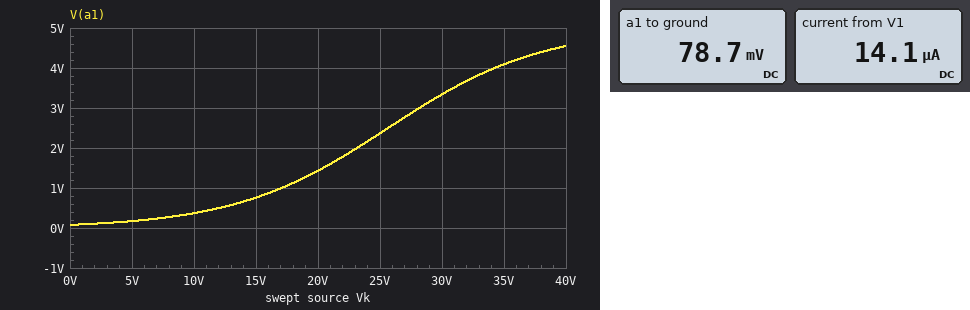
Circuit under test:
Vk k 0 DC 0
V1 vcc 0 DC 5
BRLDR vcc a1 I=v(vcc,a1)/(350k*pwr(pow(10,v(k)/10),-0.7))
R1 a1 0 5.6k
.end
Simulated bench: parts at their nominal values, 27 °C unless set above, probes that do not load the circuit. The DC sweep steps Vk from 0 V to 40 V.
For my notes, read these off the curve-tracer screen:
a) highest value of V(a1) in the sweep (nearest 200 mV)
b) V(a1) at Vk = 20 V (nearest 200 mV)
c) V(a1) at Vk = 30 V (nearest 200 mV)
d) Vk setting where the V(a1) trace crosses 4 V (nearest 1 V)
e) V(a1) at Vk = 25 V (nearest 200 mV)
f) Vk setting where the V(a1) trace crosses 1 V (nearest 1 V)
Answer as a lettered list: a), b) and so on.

a) 4.6 V
b) 1.4 V
c) 3.4 V
d) 34 V
e) 2.4 V
f) 17 V
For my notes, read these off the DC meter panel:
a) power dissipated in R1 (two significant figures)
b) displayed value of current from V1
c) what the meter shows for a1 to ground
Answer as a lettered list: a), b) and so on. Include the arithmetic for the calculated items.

a) (78.7 mV)^2 / 5.6 kΩ = 1.1 µW
b) 14.1 µA
c) 78.7 mV
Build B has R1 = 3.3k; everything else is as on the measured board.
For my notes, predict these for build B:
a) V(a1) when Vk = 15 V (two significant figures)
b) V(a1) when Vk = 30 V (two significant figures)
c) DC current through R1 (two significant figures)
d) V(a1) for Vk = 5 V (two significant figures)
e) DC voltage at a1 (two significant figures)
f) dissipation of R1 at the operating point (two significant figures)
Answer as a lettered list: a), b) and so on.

a) 480 mV
b) 2.7 V
c) 14 µA
d) 100 mV
e) 47 mV
f) 660 nW
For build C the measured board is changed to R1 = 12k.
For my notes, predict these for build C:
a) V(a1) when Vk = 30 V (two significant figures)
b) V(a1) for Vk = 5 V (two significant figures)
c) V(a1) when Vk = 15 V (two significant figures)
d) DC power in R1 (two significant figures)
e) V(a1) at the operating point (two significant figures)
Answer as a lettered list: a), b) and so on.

a) 4.1 V
b) 360 mV
c) 1.4 V
d) 2.3 µW
e) 170 mV
